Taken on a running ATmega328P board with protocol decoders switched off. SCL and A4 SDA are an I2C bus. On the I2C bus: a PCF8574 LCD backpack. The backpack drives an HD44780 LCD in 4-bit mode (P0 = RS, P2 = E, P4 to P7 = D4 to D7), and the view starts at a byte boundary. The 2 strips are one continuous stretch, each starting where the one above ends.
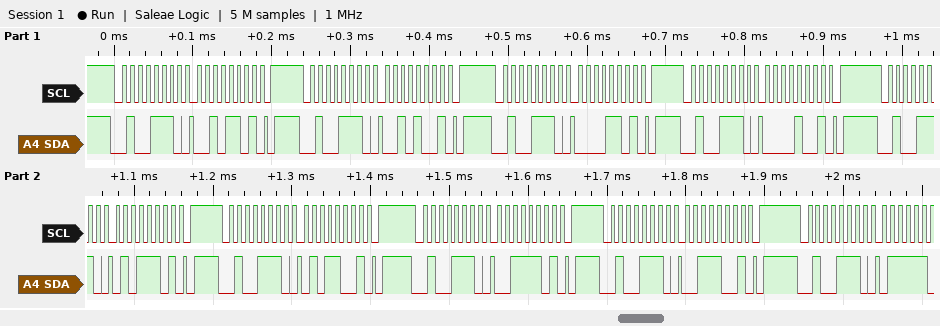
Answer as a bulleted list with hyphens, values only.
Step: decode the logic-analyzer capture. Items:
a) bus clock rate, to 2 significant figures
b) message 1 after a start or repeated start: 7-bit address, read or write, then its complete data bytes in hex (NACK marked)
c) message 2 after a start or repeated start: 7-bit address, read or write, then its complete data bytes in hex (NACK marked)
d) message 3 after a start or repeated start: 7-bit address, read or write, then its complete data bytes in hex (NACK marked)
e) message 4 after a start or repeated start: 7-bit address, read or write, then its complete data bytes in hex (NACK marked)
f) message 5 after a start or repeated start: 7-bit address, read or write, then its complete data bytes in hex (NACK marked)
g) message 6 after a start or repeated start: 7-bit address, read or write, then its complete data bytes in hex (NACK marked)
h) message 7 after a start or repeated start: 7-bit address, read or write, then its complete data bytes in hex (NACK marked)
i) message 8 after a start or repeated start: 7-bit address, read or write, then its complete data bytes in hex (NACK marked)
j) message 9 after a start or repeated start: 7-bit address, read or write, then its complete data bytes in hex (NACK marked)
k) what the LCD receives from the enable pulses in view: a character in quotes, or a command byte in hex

- 100 kHz
- 0x27 write: 2D
- 0x27 write: 29
- 0x27 write: 0D
- 0x27 write: 09
- 0x27 write: 5D
- 0x27 write: 59
- 0x27 write: 3D
- 0x27 write: 39
- 0x27 write
- ' ' 'S'
